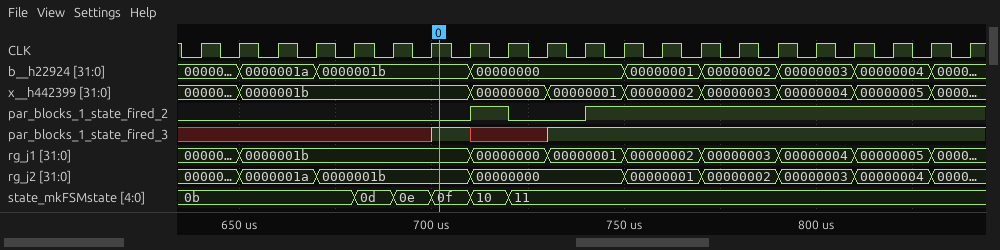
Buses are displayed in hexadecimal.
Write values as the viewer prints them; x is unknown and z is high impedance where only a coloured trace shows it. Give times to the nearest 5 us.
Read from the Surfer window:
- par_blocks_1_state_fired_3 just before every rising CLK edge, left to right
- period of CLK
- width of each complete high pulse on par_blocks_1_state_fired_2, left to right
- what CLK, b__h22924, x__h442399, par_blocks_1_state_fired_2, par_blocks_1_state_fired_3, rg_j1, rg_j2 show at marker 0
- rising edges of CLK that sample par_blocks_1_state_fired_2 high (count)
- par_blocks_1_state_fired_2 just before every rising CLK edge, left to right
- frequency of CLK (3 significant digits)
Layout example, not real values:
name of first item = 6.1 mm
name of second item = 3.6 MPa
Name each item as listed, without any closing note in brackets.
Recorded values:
par_blocks_1_state_fired_3 just before every rising CLK edge, left to right = x x x x x x x 1 x x 1 1 1 1 1 1 1 1 1 1 1
period of CLK = 10 us
width of each complete high pulse on par_blocks_1_state_fired_2, left to right = 10 us
what CLK, b__h22924, x__h442399, par_blocks_1_state_fired_2, par_blocks_1_state_fired_3, rg_j1, rg_j2 show at marker 0 = CLK=1, b__h22924=0000001b, x__h442399=0000001b, par_blocks_1_state_fired_2=0, par_blocks_1_state_fired_3=1, rg_j1=0000001b, rg_j2=0000001b
rising edges of CLK that sample par_blocks_1_state_fired_2 high = 11
par_blocks_1_state_fired_2 just before every rising CLK edge, left to right = 0 0 0 0 0 0 0 0 1 0 0 1 1 1 1 1 1 1 1 1 1
frequency of CLK = 100 kHz
